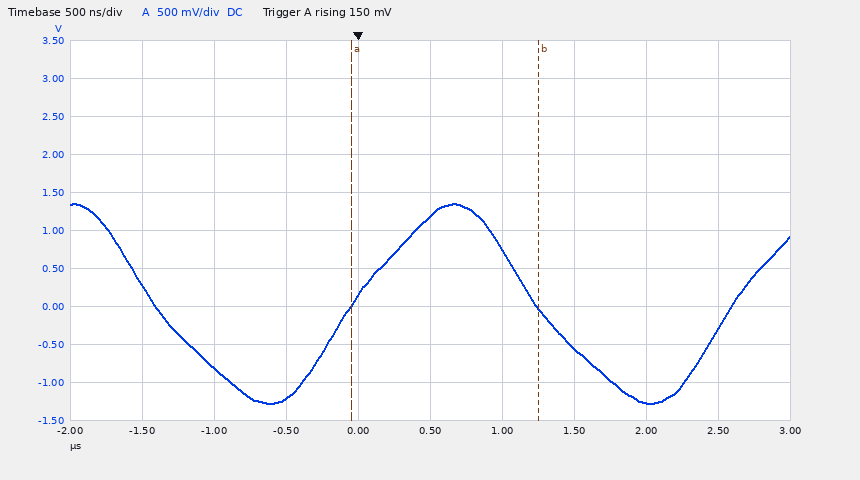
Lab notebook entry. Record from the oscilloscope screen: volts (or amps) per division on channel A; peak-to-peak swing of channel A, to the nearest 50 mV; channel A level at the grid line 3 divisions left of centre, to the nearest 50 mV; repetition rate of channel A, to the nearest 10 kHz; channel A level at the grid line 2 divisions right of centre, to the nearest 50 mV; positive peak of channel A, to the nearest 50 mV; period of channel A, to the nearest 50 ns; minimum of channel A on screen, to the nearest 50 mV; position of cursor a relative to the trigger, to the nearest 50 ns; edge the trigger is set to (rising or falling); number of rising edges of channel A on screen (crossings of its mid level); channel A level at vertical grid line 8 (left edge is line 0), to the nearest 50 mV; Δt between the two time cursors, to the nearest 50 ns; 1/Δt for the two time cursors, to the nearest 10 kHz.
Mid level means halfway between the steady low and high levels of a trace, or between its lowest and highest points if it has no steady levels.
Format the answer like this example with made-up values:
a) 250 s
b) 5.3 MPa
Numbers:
a) 500 mV
b) 2.65 V
c) -800 mV
d) 380 kHz
e) -550 mV
f) 1.35 V
g) 2.65 µs
h) -1.30 V
i) -50 ns
j) rising
k) 2
l) -1.25 V
m) 1.30 µs
n) 770 kHz
